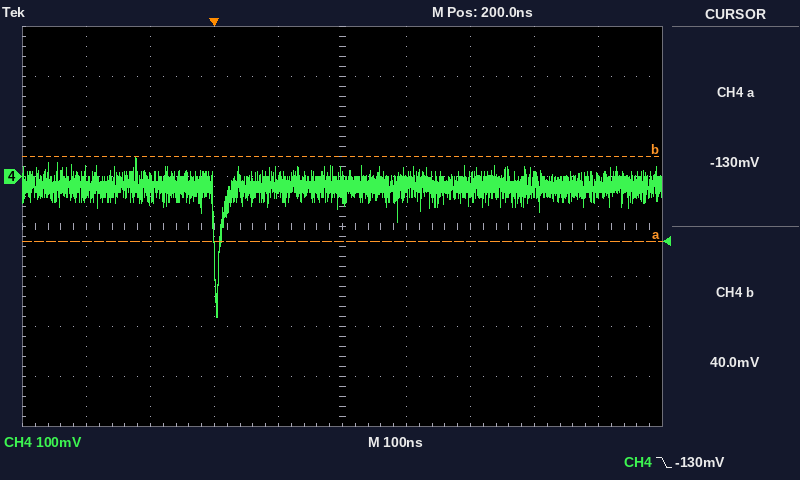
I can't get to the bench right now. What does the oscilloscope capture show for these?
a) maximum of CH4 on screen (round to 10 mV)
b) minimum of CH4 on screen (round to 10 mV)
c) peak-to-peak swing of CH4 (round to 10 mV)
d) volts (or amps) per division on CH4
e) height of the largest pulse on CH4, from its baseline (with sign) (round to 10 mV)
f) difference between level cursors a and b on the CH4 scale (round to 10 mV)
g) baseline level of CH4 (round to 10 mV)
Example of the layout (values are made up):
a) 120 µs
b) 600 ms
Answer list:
a) 40 mV
b) -280 mV
c) 320 mV
d) 100 mV
e) -260 mV
f) 170 mV
g) -20 mV
